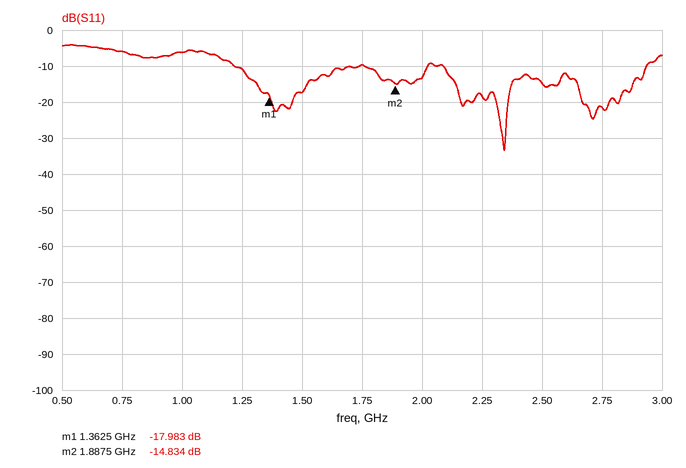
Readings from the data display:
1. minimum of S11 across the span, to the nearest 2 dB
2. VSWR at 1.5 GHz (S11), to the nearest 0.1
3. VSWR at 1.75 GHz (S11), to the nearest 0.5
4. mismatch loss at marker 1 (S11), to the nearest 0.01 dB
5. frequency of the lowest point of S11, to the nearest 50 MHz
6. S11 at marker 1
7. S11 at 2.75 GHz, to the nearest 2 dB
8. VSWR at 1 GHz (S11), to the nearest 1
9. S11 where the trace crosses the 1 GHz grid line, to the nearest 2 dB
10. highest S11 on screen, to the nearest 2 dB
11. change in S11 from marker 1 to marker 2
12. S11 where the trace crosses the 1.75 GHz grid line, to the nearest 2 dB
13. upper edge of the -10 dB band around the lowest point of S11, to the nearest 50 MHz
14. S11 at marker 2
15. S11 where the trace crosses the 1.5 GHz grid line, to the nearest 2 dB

-34 dB
1.3
2.0
0.07 dB
2.35 GHz
-17.983 dB
-22 dB
3
-6 dB
-4 dB
3.149 dB
-10 dB
2.95 GHz
-14.834 dB
-18 dB
